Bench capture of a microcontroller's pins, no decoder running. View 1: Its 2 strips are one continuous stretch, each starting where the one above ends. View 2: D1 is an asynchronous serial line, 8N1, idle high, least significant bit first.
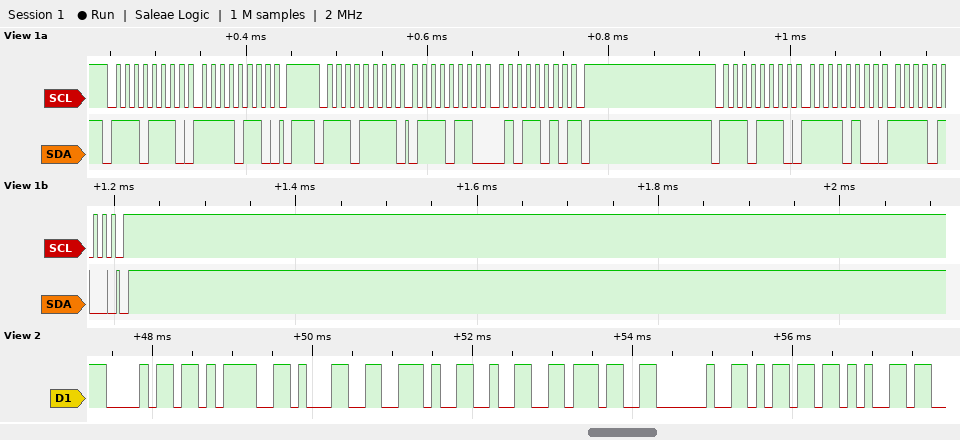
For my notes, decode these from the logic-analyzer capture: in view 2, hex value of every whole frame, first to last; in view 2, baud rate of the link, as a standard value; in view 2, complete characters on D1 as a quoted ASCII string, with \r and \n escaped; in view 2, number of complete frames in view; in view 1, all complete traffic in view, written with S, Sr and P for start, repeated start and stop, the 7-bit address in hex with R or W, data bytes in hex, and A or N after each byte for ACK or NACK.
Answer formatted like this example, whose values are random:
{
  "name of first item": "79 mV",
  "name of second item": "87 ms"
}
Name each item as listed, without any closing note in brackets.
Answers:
{
  "in view 2, hex value of every whole frame, first to last": "68 3D 31 2E 32 37 20 6D 65",
  "in view 2, baud rate of the link, as a standard value": "9600 baud",
  "in view 2, complete characters on D1 as a quoted ASCII string, with \\r and \\n escaped": "\"h=1.27 me\"",
  "in view 2, number of complete frames in view": "9",
  "in view 1, all complete traffic in view, written with S, Sr and P for start, repeated start and stop, the 7-bit address in hex with R or W, data bytes in hex, and A or N after each byte for ACK or NACK": "S 77W A F6 A P S 77R A 76 A 5A N P S 77W A F4 A F4 A P"
}
